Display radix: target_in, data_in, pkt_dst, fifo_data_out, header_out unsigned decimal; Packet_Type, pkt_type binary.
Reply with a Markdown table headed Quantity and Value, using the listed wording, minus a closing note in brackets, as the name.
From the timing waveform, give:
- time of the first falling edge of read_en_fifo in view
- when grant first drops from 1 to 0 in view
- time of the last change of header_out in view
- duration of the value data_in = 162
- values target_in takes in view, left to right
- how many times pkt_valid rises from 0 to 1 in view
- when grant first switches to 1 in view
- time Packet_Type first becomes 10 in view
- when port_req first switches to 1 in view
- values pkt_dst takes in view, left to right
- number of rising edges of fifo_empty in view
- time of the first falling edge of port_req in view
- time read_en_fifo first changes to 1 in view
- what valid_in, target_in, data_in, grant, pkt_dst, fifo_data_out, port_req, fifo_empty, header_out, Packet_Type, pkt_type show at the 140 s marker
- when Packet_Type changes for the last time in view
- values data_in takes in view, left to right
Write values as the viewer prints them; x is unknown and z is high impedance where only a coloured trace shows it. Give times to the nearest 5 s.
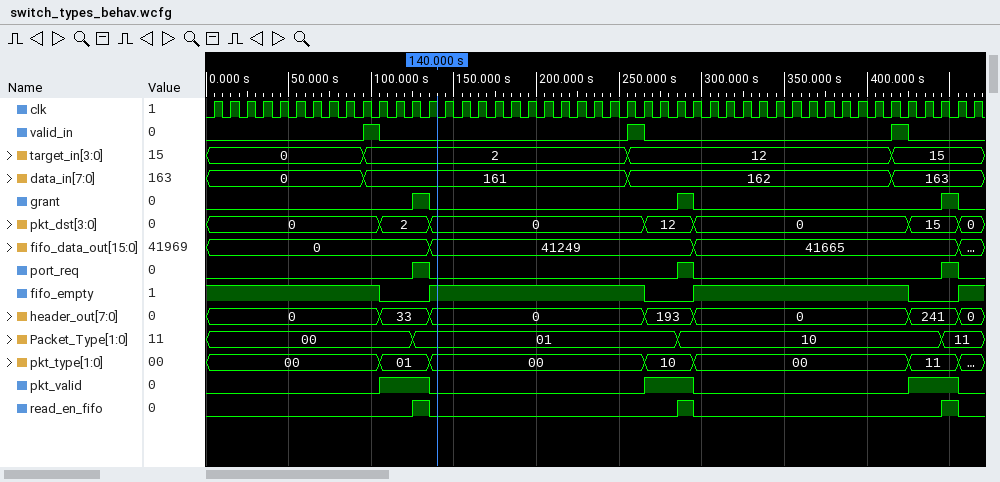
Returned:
| Quantity | Value |
|---|---|
| time of the first falling edge of read_en_fifo in view | 135 s |
| when grant first drops from 1 to 0 in view | 135 s |
| time of the last change of header_out in view | 455 s |
| duration of the value data_in = 162 | 160 s |
| values target_in takes in view, left to right | 0, 2, 12, 15 |
| how many times pkt_valid rises from 0 to 1 in view | 3 |
| when grant first switches to 1 in view | 125 s |
| time Packet_Type first becomes 10 in view | 285 s |
| when port_req first switches to 1 in view | 125 s |
| values pkt_dst takes in view, left to right | 0, 2, 0, 12, 0, 15, 0 |
| number of rising edges of fifo_empty in view | 3 |
| time of the first falling edge of port_req in view | 135 s |
| time read_en_fifo first changes to 1 in view | 125 s |
| what valid_in, target_in, data_in, grant, pkt_dst, fifo_data_out, port_req, fifo_empty, header_out, Packet_Type, pkt_type show at the 140 s marker | valid_in=0, target_in=2, data_in=161, grant=0, pkt_dst=0, fifo_data_out=41249, port_req=0, fifo_empty=1, header_out=0, Packet_Type=01, pkt_type=00 |
| when Packet_Type changes for the last time in view | 445 s |
| values data_in takes in view, left to right | 0, 161, 162, 163 |
